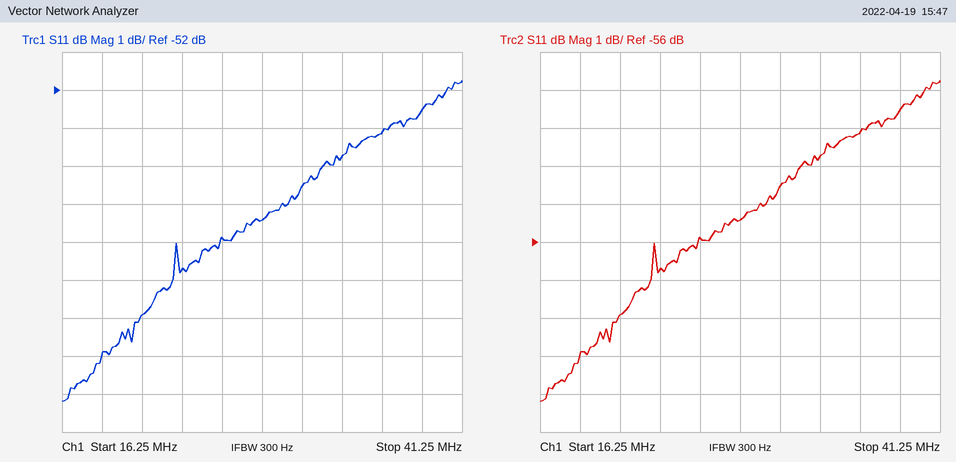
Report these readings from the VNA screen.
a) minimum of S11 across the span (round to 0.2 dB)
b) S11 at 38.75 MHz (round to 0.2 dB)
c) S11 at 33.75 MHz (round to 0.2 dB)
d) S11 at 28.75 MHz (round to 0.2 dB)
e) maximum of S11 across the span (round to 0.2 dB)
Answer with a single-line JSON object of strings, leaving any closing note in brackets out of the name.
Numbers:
{"minimum of S11 across the span": "-60.2 dB", "S11 at 38.75 MHz": "-52.6 dB", "S11 at 33.75 MHz": "-53.8 dB", "S11 at 28.75 MHz": "-55.4 dB", "maximum of S11 across the span": "-51.8 dB"}
